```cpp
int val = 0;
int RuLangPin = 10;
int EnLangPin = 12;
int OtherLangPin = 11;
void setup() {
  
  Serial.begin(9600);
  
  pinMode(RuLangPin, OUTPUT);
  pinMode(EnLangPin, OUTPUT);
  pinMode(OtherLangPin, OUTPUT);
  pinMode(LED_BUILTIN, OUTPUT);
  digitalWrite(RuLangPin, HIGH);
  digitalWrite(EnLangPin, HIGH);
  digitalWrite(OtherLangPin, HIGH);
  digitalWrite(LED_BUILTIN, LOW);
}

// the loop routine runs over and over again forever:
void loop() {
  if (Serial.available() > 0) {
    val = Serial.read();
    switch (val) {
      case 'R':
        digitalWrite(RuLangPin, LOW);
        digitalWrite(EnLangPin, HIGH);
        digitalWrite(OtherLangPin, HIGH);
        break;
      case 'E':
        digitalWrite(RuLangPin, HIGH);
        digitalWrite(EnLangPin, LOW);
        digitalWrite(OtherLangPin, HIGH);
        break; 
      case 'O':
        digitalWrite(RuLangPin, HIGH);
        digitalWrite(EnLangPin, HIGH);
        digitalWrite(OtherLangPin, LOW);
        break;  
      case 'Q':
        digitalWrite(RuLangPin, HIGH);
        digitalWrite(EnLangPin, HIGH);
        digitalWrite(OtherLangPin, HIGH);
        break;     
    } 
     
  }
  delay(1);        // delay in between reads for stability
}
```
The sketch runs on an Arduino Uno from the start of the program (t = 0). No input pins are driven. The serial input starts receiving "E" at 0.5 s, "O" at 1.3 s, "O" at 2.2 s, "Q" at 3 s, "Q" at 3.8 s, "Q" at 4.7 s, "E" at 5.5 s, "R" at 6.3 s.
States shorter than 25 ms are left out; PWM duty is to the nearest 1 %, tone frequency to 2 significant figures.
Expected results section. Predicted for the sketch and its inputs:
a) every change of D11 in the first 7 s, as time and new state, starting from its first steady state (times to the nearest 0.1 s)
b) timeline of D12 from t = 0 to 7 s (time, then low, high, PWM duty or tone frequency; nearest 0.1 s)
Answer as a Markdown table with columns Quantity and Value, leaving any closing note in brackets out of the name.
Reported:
| Quantity | Value |
|---|---|
| every change of D11 in the first 7 s, as time and new state, starting from its first steady state | 0 s high; 1.3 s low; 3 s high |
| timeline of D12 from t = 0 to 7 s | 0 s high; 0.5 s low; 1.3 s high; 5.5 s low; 6.3 s high |
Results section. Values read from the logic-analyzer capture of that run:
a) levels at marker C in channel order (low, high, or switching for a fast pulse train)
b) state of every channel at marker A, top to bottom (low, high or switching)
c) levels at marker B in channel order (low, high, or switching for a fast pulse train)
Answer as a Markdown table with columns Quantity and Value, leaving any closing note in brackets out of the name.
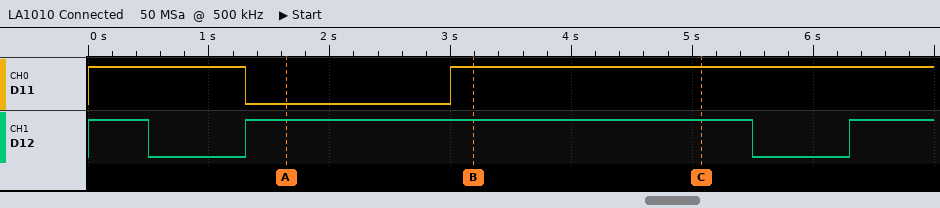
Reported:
| Quantity | Value |
|---|---|
| levels at marker C in channel order | D11 high, D12 high |
| state of every channel at marker A, top to bottom | D11 low, D12 high |
| levels at marker B in channel order | D11 high, D12 high |
